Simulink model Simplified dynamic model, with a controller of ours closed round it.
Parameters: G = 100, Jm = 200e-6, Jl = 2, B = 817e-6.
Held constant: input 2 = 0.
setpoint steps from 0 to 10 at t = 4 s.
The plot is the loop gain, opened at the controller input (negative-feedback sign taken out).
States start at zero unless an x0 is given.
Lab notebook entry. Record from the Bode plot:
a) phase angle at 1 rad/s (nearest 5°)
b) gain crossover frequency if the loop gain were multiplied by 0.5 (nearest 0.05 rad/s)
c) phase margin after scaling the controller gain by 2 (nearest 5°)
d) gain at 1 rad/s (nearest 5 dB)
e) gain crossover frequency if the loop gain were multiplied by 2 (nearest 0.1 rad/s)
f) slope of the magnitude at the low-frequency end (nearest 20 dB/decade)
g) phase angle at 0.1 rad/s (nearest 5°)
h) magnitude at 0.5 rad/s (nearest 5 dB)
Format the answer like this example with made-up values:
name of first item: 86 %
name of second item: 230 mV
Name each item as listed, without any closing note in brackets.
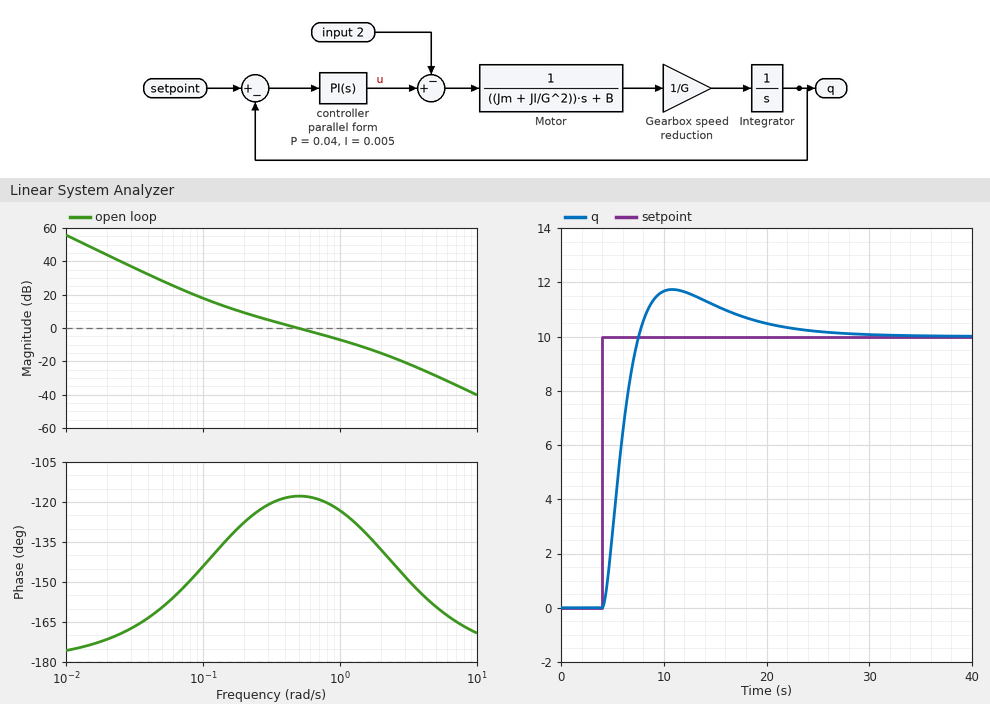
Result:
phase angle at 1 rad/s: -125°
gain crossover frequency if the loop gain were multiplied by 0.5: 0.25 rad/s
phase margin after scaling the controller gain by 2: 60°
gain at 1 rad/s: -5 dB
gain crossover frequency if the loop gain were multiplied by 2: 0.9 rad/s
slope of the magnitude at the low-frequency end: -40 dB/decade
phase angle at 0.1 rad/s: -145°
magnitude at 0.5 rad/s: 0 dB
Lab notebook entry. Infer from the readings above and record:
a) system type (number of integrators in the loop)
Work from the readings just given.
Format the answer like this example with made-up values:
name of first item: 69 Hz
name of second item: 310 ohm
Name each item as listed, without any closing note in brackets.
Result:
system type: 2
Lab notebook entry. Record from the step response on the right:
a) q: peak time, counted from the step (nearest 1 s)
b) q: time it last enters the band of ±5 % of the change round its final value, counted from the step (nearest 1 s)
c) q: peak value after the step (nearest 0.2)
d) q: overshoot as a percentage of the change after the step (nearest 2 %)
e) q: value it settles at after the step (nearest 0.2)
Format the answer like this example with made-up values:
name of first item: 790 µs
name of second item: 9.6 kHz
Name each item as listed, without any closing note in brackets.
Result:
q: peak time, counted from the step: 7 s
q: time it last enters the band of ±5 % of the change round its final value, counted from the step: 16 s
q: peak value after the step: 11.8
q: overshoot as a percentage of the change after the step: 18 %
q: value it settles at after the step: 10.0
